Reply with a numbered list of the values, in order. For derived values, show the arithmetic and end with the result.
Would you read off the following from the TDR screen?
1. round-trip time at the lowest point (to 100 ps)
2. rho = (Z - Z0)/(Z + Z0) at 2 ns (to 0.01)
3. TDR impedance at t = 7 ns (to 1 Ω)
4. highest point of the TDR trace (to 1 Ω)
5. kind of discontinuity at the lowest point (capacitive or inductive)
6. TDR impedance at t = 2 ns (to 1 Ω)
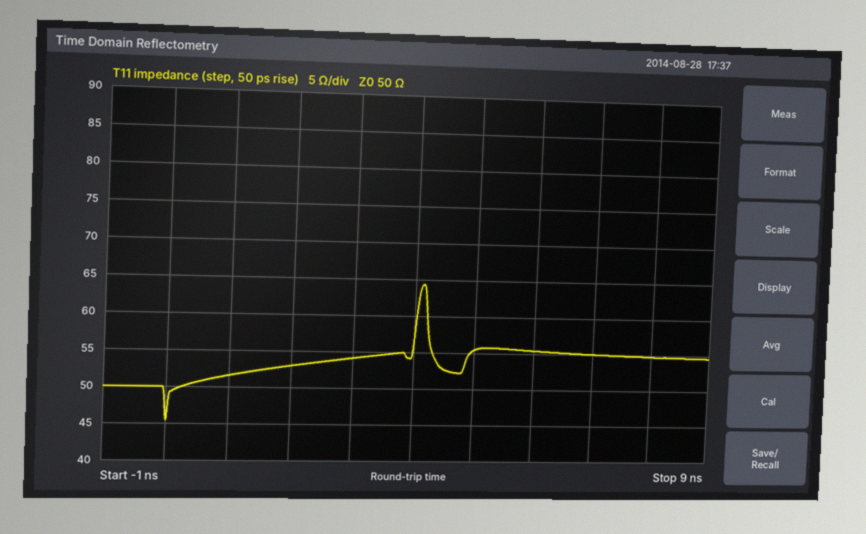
1. 0.0 ns
2. (53 − 50)/(53 + 50) ≈ +0.03
3. 55 Ω
4. 64 Ω
5. capacitive
6. 53 Ω
